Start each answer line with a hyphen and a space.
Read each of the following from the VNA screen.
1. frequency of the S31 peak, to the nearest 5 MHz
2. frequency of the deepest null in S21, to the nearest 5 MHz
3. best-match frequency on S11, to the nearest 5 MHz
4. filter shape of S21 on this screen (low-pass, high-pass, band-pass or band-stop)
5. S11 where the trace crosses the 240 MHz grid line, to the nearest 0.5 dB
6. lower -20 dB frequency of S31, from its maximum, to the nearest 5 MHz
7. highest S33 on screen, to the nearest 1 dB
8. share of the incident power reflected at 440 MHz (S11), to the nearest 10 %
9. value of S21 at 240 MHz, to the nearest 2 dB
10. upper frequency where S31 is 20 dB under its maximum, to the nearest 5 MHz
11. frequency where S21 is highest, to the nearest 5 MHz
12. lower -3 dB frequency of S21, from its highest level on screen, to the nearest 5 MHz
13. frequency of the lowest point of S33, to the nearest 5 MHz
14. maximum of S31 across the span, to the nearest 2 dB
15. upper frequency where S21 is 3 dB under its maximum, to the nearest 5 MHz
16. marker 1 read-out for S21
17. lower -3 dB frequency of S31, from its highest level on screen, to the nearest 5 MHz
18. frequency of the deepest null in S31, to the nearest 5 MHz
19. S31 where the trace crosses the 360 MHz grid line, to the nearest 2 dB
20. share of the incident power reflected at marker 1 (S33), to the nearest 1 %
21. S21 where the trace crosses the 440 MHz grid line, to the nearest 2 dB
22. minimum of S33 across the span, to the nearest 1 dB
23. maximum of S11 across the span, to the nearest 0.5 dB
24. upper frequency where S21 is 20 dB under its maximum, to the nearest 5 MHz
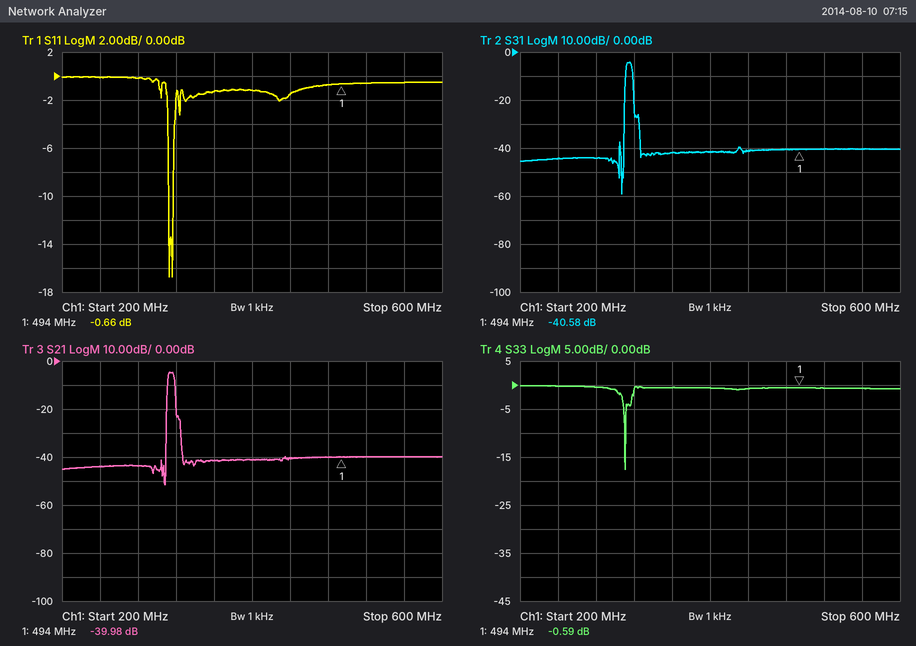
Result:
- 315 MHz
- 310 MHz
- 315 MHz
- band-pass
- 0.0 dB
- 310 MHz
- 0 dB
- 70 %
- -44 dB
- 320 MHz
- 315 MHz
- 310 MHz
- 310 MHz
- -4 dB
- 320 MHz
- -39.98 dB
- 310 MHz
- 305 MHz
- -42 dB
- 87 %
- -40 dB
- -18 dB
- 0.0 dB
- 325 MHz
